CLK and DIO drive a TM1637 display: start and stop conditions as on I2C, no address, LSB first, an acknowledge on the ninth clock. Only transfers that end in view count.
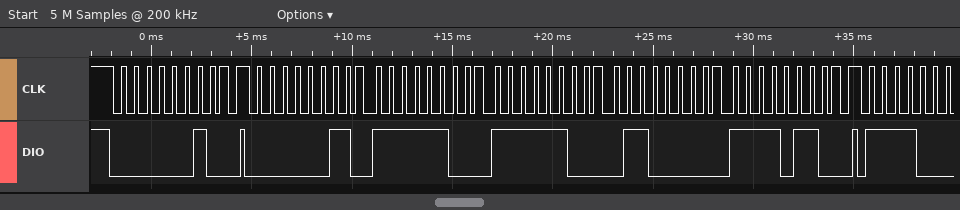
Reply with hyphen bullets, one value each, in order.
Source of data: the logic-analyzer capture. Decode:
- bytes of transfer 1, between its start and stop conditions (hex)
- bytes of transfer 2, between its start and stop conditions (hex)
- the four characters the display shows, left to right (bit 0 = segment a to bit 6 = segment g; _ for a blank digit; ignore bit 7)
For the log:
- 40
- C0 3F 3F 06 6F
- 0019
